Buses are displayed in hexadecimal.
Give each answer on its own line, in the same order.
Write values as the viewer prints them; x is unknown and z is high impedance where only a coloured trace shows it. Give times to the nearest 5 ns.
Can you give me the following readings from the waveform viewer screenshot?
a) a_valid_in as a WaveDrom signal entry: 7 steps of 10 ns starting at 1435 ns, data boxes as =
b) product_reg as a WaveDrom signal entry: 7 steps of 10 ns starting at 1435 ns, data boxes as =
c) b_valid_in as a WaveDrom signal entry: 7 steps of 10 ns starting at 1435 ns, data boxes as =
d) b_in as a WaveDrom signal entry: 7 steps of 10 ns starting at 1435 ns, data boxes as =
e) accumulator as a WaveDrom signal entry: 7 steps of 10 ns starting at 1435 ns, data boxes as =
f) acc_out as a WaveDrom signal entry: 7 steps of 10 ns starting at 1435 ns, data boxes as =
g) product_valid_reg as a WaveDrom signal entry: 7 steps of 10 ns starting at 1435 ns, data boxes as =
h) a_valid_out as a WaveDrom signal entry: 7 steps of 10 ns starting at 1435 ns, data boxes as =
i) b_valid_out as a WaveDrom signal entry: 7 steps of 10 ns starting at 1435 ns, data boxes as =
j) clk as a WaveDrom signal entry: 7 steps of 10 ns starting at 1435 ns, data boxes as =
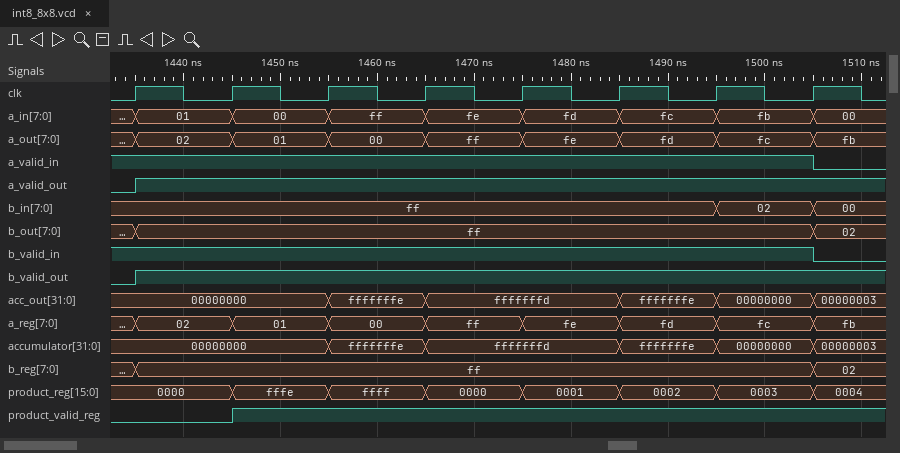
{name: 'a_valid_in', wave: '1......'}
{name: 'product_reg', wave: '=======', data: '0000 fffe ffff 0000 0001 0002 0003'}
{name: 'b_valid_in', wave: '1......'}
{name: 'b_in', wave: '=.....=', data: 'ff 02'}
{name: 'accumulator', wave: '=.==.==', data: '00000000 fffffffe fffffffd fffffffe 00000000'}
{name: 'acc_out', wave: '=.==.==', data: '00000000 fffffffe fffffffd fffffffe 00000000'}
{name: 'product_valid_reg', wave: '01.....'}
{name: 'a_valid_out', wave: '1......'}
{name: 'b_valid_out', wave: '1......'}
{name: 'clk', wave: 'p......'}
